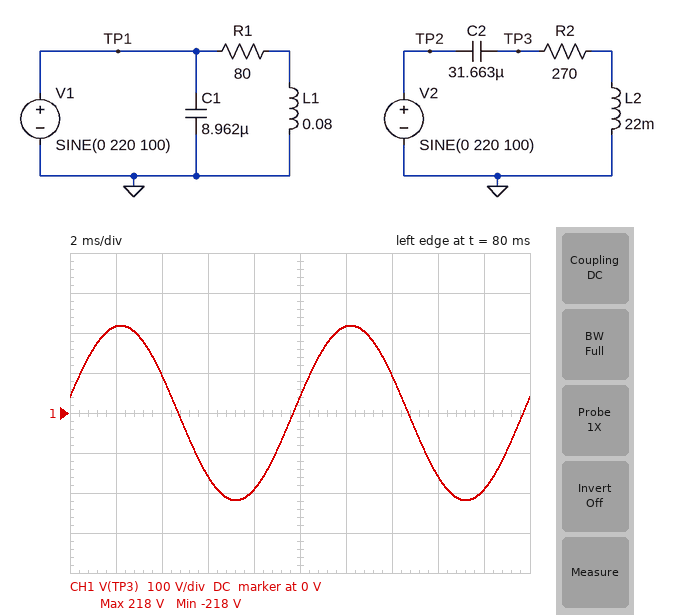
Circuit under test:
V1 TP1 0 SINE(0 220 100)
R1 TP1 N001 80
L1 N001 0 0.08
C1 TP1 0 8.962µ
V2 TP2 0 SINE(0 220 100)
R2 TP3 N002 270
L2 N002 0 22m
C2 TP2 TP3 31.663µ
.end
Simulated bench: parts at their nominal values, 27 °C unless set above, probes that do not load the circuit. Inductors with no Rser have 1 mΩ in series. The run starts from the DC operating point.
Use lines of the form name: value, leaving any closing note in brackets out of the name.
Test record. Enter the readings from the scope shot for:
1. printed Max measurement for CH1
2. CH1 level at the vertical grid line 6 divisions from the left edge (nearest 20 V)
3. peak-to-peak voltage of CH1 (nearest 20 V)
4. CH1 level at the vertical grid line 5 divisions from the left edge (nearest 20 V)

printed Max measurement for CH1: 218 V
CH1 level at the vertical grid line 6 divisions from the left edge: 220 V
peak-to-peak voltage of CH1: 440 V
CH1 level at the vertical grid line 5 divisions from the left edge: 40 V
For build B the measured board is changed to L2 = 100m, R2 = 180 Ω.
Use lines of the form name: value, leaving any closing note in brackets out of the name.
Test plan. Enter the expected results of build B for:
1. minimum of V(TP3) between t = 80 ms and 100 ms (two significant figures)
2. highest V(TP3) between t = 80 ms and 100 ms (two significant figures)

minimum of V(TP3) between t = 80 ms and 100 ms: -230 V
highest V(TP3) between t = 80 ms and 100 ms: 230 V
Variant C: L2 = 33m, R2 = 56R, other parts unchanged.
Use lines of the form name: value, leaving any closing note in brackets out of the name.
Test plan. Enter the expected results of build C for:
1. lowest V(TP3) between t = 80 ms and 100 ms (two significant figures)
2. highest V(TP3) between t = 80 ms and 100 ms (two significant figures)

lowest V(TP3) between t = 80 ms and 100 ms: -210 V
highest V(TP3) between t = 80 ms and 100 ms: 210 V
